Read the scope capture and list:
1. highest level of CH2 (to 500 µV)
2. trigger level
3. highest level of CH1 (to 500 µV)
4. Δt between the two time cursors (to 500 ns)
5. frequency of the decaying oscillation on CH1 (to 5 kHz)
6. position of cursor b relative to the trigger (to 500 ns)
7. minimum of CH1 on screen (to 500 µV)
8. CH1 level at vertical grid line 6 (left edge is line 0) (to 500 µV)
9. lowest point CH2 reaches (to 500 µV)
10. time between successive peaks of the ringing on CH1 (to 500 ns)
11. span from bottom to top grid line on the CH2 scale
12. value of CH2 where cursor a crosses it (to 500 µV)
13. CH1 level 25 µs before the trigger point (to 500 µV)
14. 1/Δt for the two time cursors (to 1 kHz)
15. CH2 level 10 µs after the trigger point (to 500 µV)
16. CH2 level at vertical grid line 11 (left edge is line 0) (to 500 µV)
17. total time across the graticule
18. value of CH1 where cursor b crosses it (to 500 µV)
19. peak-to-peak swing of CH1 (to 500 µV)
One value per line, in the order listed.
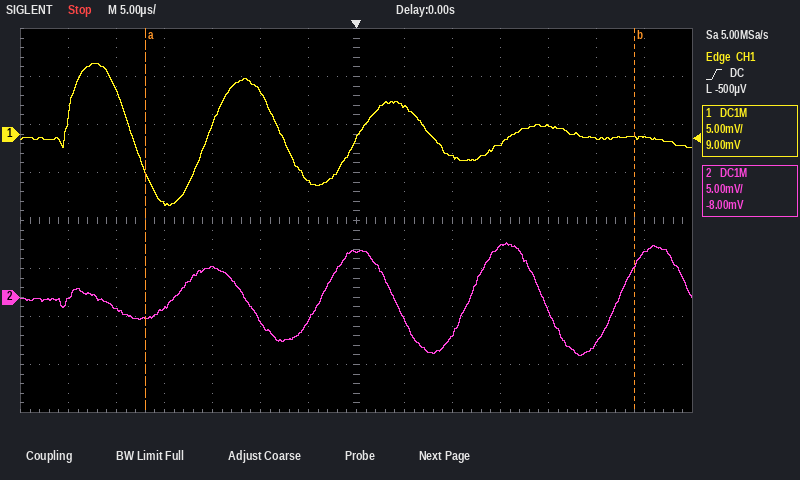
5.5 mV
-500 µV
7.5 mV
51.0 µs
65 kHz
+29.0 µs
-7.5 mV
-5.0 mV
-6.0 mV
15.5 µs
40 mV
-2.0 mV
4.5 mV
20 kHz
-4.0 mV
-1.5 mV
70 µs
-500 µV
15.0 mV
